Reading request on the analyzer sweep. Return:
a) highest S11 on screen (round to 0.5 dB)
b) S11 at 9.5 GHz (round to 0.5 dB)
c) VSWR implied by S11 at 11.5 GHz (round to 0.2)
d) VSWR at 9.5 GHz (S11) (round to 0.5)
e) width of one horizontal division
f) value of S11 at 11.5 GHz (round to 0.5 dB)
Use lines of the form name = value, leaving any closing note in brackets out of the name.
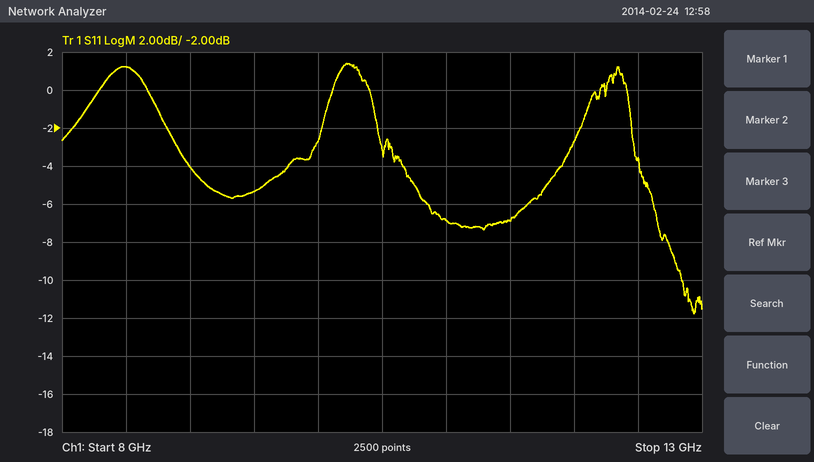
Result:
highest S11 on screen = 1.5 dB
S11 at 9.5 GHz = -5.5 dB
VSWR implied by S11 at 11.5 GHz = 2.6
VSWR at 9.5 GHz (S11) = 3.5
width of one horizontal division = 500 MHz
value of S11 at 11.5 GHz = -7.0 dB
